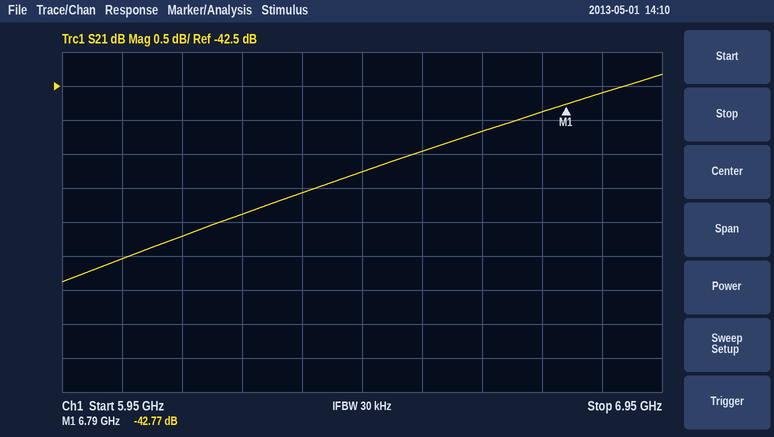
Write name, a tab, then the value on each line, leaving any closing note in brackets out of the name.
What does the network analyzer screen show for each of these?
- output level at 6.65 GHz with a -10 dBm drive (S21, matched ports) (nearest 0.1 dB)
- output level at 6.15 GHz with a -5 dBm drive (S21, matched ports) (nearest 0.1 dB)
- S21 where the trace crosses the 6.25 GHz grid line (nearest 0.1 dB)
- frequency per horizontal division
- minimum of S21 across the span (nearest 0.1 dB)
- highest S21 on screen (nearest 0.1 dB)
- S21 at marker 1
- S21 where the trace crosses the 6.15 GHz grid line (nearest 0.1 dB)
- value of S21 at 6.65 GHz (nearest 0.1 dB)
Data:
output level at 6.65 GHz with a -10 dBm drive (S21, matched ports)	-53.2 dBm
output level at 6.15 GHz with a -5 dBm drive (S21, matched ports)	-49.7 dBm
S21 where the trace crosses the 6.25 GHz grid line	-44.4 dB
frequency per horizontal division	100 MHz
minimum of S21 across the span	-45.4 dB
highest S21 on screen	-42.3 dB
S21 at marker 1	-42.77 dB
S21 where the trace crosses the 6.15 GHz grid line	-44.7 dB
value of S21 at 6.65 GHz	-43.2 dB
